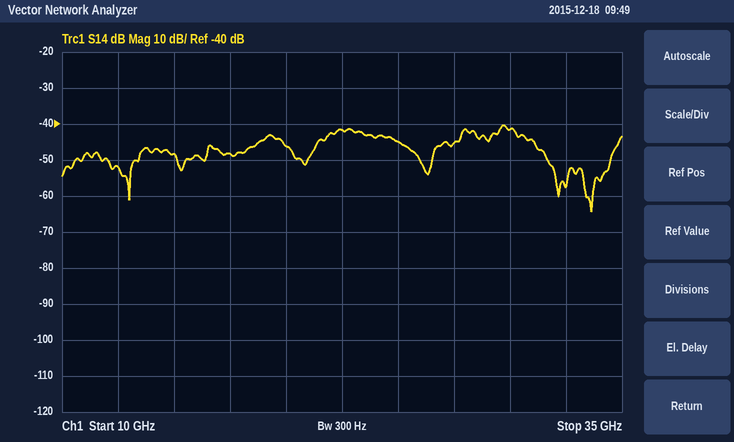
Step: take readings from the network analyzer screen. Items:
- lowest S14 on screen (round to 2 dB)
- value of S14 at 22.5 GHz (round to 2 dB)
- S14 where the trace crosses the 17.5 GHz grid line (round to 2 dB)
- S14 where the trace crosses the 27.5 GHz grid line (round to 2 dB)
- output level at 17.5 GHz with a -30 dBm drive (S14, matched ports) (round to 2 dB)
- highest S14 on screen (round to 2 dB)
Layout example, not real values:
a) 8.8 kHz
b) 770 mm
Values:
a) -64 dB
b) -42 dB
c) -48 dB
d) -46 dB
e) -78 dBm
f) -40 dB
